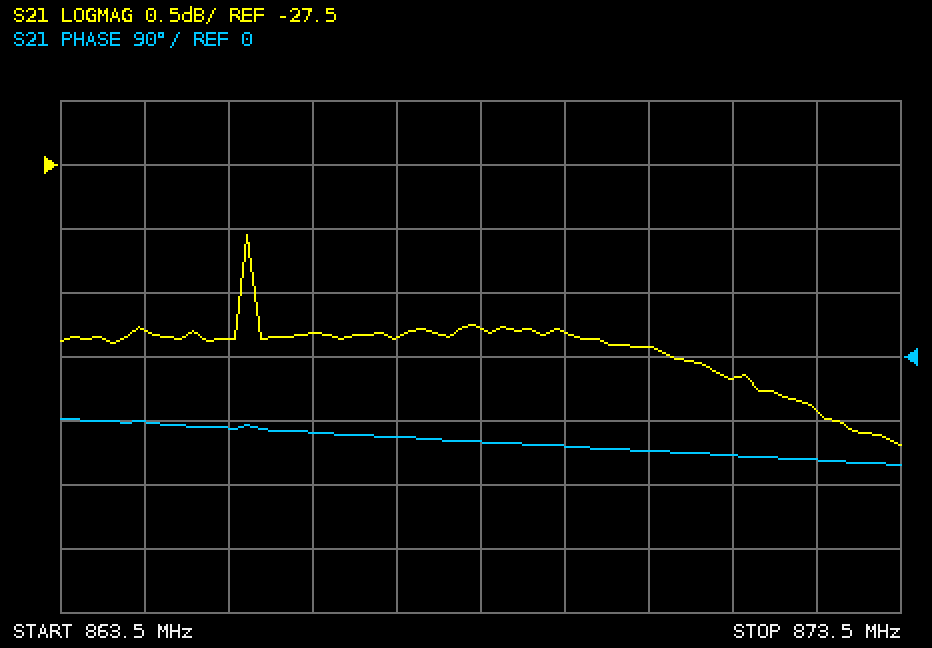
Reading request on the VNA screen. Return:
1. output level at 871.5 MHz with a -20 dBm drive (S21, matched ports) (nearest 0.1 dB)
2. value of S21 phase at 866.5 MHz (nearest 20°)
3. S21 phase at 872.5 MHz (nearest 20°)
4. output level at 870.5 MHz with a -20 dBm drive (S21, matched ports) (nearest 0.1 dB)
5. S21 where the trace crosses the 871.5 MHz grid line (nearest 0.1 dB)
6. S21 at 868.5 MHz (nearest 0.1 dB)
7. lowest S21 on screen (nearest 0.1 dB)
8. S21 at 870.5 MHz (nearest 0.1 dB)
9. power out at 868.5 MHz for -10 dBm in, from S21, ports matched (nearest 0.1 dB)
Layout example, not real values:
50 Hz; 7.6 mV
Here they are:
-49.2 dBm; -100°; -140°; -48.9 dBm; -29.2 dB; -28.8 dB; -29.7 dB; -28.9 dB; -38.8 dBm
